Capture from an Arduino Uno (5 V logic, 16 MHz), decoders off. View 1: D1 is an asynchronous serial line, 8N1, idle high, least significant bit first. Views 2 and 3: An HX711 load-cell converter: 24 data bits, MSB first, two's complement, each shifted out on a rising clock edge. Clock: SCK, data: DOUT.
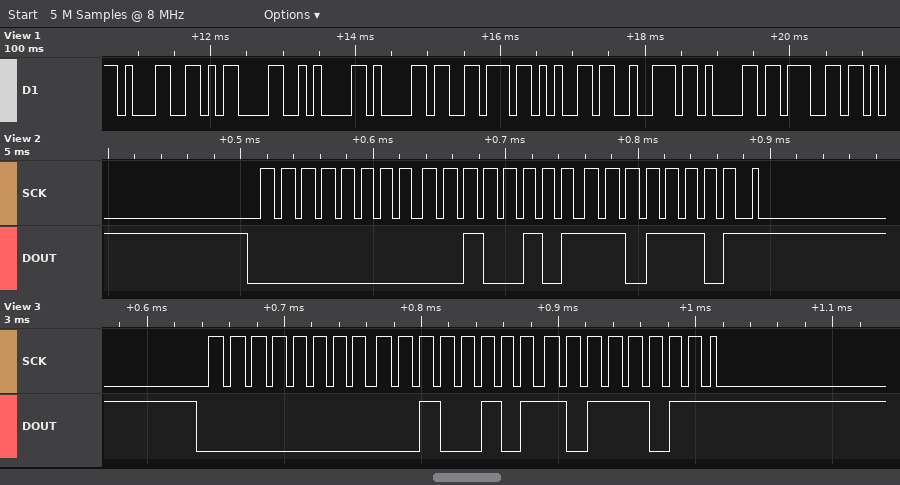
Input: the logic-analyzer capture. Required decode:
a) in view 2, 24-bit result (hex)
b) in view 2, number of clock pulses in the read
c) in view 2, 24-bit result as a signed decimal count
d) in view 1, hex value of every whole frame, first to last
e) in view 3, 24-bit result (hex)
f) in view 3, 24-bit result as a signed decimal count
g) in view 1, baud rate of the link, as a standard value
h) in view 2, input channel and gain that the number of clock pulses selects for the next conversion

0x0025DD
25
9693
31 0D 0A 61 76 65 72 61 67
0x0025BB
9659
9600 baud
channel A, gain 128
